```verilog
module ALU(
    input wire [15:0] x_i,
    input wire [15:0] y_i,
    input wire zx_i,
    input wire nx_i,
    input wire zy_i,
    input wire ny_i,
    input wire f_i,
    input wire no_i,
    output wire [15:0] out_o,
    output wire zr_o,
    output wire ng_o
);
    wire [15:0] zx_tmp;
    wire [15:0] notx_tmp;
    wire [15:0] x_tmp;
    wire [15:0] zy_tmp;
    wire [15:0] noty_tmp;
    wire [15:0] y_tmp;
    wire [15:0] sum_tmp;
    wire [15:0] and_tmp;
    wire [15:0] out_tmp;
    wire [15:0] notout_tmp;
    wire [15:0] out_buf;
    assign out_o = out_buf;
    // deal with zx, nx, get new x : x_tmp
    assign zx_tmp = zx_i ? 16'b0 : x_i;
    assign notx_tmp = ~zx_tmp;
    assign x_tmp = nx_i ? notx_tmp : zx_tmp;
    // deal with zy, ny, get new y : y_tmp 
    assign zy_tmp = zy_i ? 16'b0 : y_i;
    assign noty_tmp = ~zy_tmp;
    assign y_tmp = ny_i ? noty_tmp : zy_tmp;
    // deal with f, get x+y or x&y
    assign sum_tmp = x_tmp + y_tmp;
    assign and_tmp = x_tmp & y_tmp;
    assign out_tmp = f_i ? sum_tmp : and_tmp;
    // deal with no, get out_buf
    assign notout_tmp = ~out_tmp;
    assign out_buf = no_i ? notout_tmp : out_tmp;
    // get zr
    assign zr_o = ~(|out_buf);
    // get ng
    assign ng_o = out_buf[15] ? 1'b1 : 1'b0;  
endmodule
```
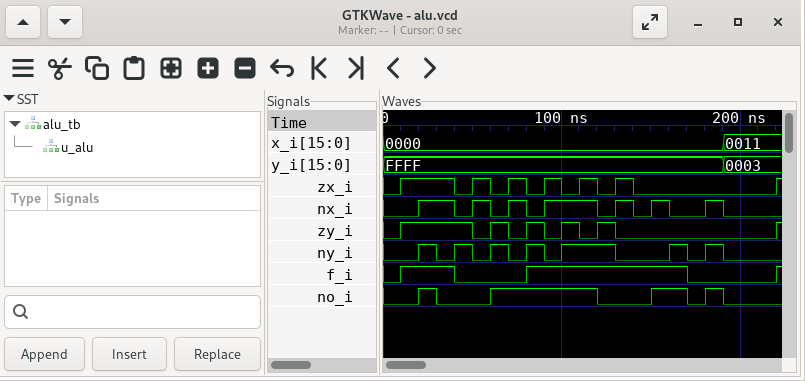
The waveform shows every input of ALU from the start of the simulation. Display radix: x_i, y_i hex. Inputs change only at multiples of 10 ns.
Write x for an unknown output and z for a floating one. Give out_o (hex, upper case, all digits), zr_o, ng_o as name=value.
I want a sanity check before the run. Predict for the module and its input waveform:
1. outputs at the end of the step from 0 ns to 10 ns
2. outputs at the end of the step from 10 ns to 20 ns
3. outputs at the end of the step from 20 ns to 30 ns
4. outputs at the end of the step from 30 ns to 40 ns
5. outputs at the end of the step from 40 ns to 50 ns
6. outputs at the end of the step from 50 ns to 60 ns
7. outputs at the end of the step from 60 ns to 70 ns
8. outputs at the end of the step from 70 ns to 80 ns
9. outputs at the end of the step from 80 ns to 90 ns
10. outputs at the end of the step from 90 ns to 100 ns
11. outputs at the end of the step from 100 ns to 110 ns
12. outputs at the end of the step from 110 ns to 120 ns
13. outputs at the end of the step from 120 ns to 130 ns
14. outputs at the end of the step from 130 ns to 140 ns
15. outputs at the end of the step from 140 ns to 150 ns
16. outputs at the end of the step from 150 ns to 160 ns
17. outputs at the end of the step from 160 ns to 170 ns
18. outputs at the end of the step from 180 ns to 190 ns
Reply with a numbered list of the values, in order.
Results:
1. out_o=0000, zr_o=1, ng_o=0
2. out_o=0000, zr_o=1, ng_o=0
3. out_o=0001, zr_o=0, ng_o=0
4. out_o=FFFF, zr_o=0, ng_o=1
5. out_o=0000, zr_o=1, ng_o=0
6. out_o=FFFF, zr_o=0, ng_o=1
7. out_o=FFFF, zr_o=0, ng_o=1
8. out_o=0000, zr_o=1, ng_o=0
9. out_o=0000, zr_o=1, ng_o=0
10. out_o=0001, zr_o=0, ng_o=0
11. out_o=0001, zr_o=0, ng_o=0
12. out_o=0000, zr_o=1, ng_o=0
13. out_o=FFFF, zr_o=0, ng_o=1
14. out_o=FFFE, zr_o=0, ng_o=1
15. out_o=FFFF, zr_o=0, ng_o=1
16. out_o=0001, zr_o=0, ng_o=0
17. out_o=FFFF, zr_o=0, ng_o=1
18. out_o=FFFF, zr_o=0, ng_o=1
